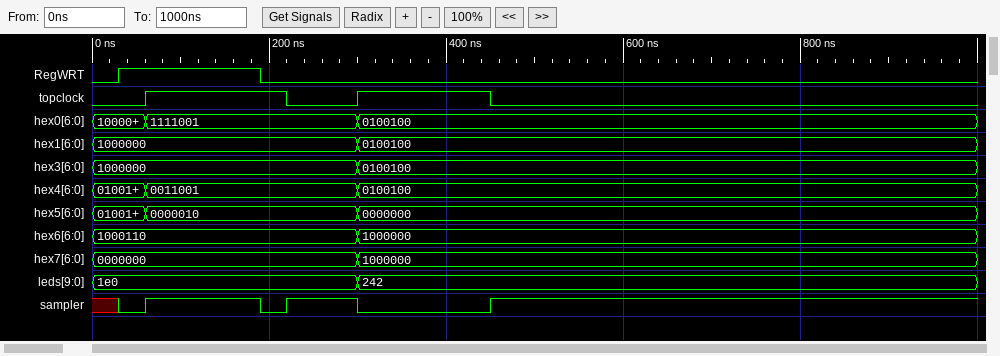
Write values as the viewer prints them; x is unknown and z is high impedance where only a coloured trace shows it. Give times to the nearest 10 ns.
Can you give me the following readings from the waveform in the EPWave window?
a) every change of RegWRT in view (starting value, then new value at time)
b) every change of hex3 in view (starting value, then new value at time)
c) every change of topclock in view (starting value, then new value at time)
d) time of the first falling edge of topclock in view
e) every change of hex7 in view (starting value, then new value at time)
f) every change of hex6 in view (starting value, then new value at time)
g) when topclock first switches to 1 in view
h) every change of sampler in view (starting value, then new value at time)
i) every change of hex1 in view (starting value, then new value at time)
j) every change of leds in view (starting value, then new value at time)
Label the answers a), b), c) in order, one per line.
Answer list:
a) 0, 1 at 30 ns, 0 at 190 ns
b) 1000000, 0100100 at 300 ns
c) 0, 1 at 60 ns, 0 at 220 ns, 1 at 300 ns, 0 at 450 ns
d) 220 ns
e) 0000000, 1000000 at 300 ns
f) 1000110, 1000000 at 300 ns
g) 60 ns
h) x, 0 at 30 ns, 1 at 60 ns, 0 at 190 ns, 1 at 220 ns, 0 at 300 ns, 1 at 450 ns
i) 1000000, 0100100 at 300 ns
j) 1e0, 242 at 300 ns
